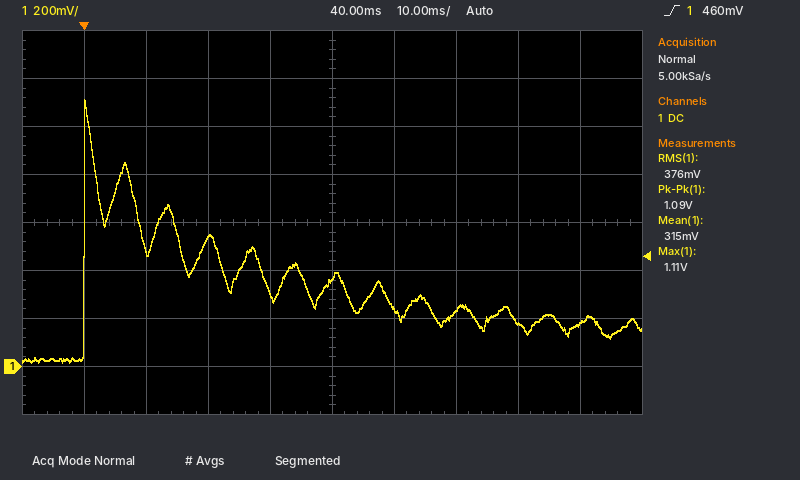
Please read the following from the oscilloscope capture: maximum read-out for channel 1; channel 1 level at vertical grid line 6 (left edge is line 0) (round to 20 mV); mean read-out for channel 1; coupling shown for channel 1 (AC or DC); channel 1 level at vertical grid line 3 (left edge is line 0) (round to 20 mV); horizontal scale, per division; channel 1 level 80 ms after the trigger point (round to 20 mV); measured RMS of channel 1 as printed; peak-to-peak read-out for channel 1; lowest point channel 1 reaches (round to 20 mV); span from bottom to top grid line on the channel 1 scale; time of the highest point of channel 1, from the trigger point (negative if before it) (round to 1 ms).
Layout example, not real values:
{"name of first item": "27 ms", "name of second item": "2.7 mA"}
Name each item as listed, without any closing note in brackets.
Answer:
{"maximum read-out for channel 1": "1.11 V", "channel 1 level at vertical grid line 6 (left edge is line 0)": "240 mV", "mean read-out for channel 1": "315 mV", "coupling shown for channel 1": "DC", "channel 1 level at vertical grid line 3 (left edge is line 0)": "540 mV", "horizontal scale, per division": "10 ms", "channel 1 level 80 ms after the trigger point": "180 mV", "measured RMS of channel 1 as printed": "376 mV", "peak-to-peak read-out for channel 1": "1.09 V", "lowest point channel 1 reaches": "20 mV", "span from bottom to top grid line on the channel 1 scale": "1.6 V", "time of the highest point of channel 1, from the trigger point (negative if before it)": "0 ms"}
